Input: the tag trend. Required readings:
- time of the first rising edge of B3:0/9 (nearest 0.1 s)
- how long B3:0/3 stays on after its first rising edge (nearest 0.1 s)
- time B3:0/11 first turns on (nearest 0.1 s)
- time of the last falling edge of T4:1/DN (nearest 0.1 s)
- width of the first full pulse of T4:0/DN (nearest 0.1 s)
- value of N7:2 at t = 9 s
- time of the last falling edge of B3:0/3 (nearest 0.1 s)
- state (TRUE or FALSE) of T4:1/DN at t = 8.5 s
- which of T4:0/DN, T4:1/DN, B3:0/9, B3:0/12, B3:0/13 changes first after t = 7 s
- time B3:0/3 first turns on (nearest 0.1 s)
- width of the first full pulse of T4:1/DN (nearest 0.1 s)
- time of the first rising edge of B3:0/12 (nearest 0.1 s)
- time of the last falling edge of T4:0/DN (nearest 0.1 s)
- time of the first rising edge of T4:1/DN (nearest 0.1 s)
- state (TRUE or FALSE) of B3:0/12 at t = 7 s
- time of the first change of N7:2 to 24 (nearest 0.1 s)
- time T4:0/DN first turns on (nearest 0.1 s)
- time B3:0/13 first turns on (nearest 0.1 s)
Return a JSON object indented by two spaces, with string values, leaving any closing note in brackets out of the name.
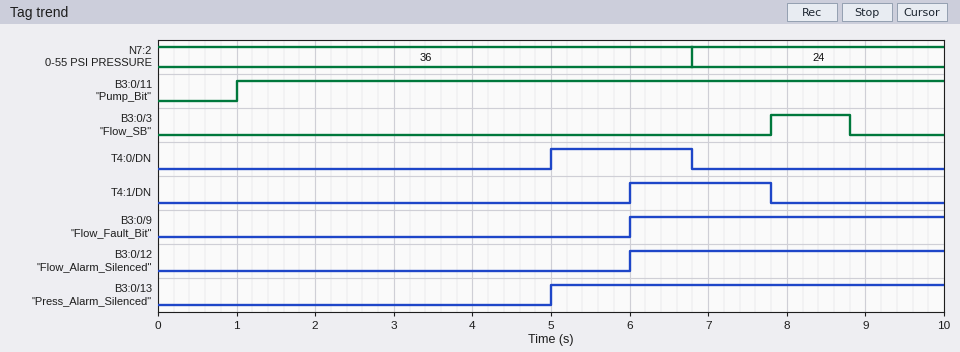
{
  "time of the first rising edge of B3:0/9": "6.0 s",
  "how long B3:0/3 stays on after its first rising edge": "1.0 s",
  "time B3:0/11 first turns on": "1.0 s",
  "time of the last falling edge of T4:1/DN": "7.8 s",
  "width of the first full pulse of T4:0/DN": "1.8 s",
  "value of N7:2 at t = 9 s": "24",
  "time of the last falling edge of B3:0/3": "8.8 s",
  "state (TRUE or FALSE) of T4:1/DN at t = 8.5 s": "FALSE",
  "which of T4:0/DN, T4:1/DN, B3:0/9, B3:0/12, B3:0/13 changes first after t = 7 s": "T4:1/DN",
  "time B3:0/3 first turns on": "7.8 s",
  "width of the first full pulse of T4:1/DN": "1.8 s",
  "time of the first rising edge of B3:0/12": "6.0 s",
  "time of the last falling edge of T4:0/DN": "6.8 s",
  "time of the first rising edge of T4:1/DN": "6.0 s",
  "state (TRUE or FALSE) of B3:0/12 at t = 7 s": "TRUE",
  "time of the first change of N7:2 to 24": "6.8 s",
  "time T4:0/DN first turns on": "5.0 s",
  "time B3:0/13 first turns on": "5.0 s"
}
